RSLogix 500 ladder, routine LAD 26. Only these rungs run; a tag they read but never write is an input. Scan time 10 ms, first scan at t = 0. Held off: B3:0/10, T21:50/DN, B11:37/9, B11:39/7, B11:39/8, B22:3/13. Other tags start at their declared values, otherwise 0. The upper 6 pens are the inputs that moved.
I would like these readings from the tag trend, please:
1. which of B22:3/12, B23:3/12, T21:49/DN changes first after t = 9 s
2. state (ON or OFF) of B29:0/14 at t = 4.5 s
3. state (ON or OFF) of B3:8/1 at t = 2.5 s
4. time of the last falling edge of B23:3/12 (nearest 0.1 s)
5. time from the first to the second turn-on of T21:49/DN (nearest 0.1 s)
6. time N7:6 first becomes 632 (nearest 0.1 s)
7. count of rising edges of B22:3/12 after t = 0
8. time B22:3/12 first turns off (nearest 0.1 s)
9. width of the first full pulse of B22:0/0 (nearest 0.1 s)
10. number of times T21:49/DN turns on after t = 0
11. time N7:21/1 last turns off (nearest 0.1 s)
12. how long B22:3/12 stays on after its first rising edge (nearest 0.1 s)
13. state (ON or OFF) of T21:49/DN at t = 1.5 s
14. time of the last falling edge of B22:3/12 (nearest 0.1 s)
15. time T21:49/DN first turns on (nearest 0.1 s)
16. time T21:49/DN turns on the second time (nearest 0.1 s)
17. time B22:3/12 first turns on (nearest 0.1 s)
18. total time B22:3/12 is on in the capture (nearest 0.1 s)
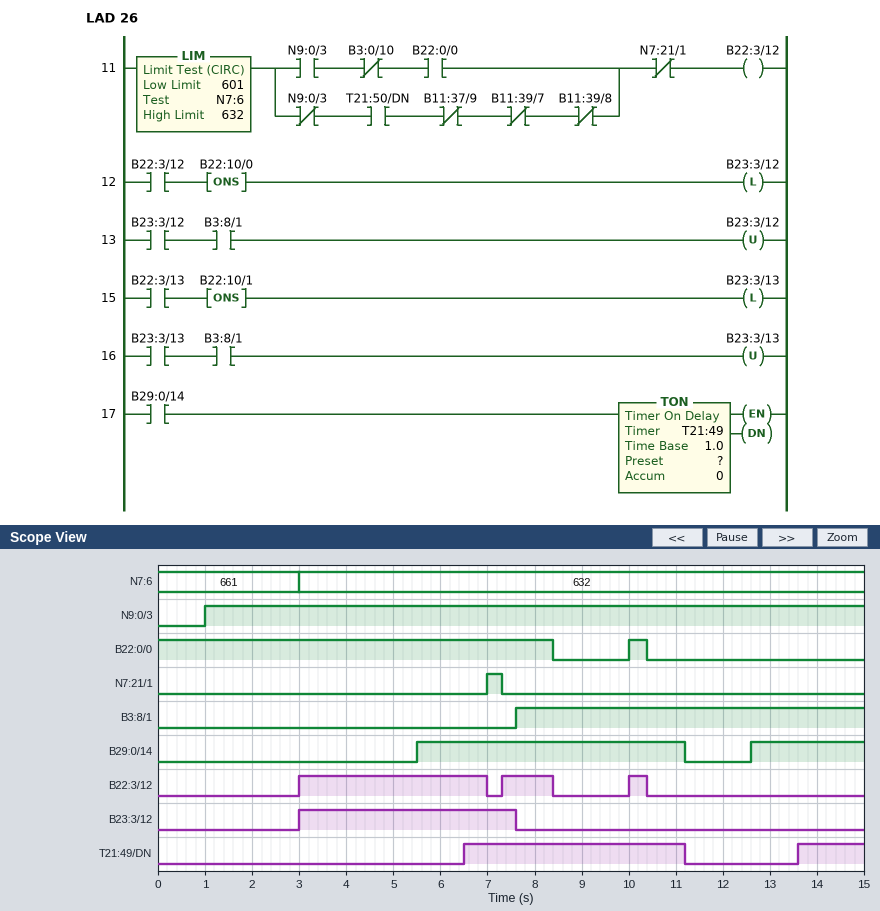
B22:3/12
OFF
OFF
7.6 s
7.1 s
3.0 s
3
7.0 s
0.4 s
2
7.3 s
4.0 s
OFF
10.4 s
6.5 s
13.6 s
3.0 s
5.5 s
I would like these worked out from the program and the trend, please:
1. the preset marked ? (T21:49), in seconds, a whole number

1 s
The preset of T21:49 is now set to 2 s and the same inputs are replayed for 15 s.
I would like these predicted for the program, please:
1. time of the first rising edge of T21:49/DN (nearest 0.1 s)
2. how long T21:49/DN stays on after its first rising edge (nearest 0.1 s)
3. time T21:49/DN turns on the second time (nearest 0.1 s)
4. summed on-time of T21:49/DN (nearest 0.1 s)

7.5 s
3.7 s
14.6 s
4.1 s
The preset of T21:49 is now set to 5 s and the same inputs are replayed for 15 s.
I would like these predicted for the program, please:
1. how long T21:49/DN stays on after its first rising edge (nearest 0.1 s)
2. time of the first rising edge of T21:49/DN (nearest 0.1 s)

0.7 s
10.5 s
